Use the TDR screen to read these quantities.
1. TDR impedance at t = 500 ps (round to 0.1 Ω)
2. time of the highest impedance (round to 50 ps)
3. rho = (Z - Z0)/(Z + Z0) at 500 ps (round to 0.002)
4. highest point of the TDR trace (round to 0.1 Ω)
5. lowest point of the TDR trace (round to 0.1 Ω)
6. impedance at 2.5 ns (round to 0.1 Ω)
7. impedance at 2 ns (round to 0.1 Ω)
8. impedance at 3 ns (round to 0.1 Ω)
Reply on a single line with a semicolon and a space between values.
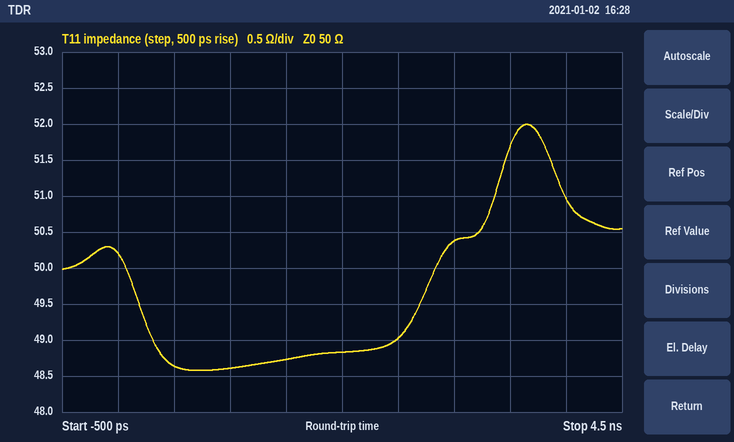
48.6 Ω; 3.65 ns; -0.014; 52.0 Ω; 48.6 Ω; 49.0 Ω; 48.8 Ω; 50.4 Ω
